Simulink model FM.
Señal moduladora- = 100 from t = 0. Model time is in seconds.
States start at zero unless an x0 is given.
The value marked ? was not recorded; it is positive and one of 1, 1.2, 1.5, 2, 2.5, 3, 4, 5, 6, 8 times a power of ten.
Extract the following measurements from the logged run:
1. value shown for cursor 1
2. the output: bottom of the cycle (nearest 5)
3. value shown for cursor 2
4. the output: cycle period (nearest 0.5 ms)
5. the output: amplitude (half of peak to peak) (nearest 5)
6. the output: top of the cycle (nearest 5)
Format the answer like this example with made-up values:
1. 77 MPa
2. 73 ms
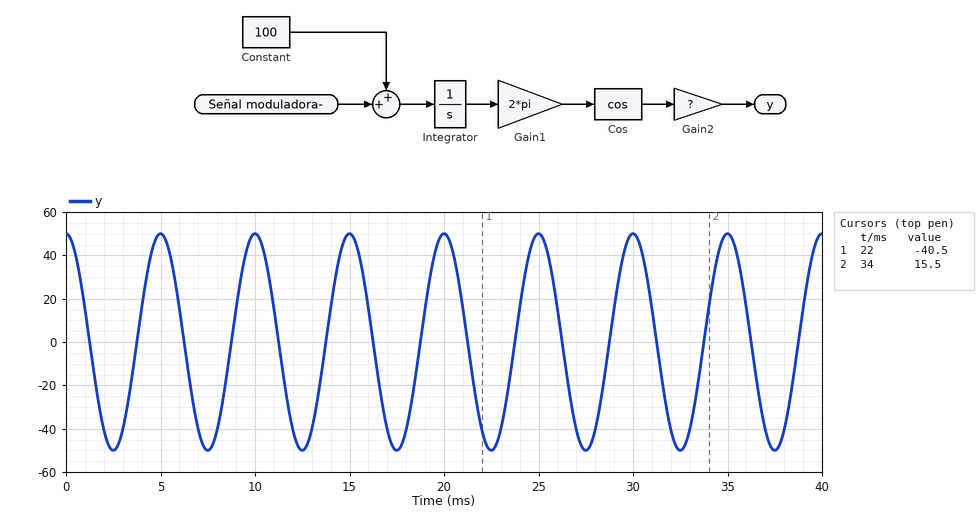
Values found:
1. -40.5
2. -50
3. 15.5
4. 5.0 ms
5. 50
6. 50
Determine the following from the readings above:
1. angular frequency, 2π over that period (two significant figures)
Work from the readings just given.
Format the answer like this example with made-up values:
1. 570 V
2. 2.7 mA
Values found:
1. 1.3 rad/ms
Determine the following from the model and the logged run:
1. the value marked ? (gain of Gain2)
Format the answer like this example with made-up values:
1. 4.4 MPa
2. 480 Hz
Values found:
1. 50
